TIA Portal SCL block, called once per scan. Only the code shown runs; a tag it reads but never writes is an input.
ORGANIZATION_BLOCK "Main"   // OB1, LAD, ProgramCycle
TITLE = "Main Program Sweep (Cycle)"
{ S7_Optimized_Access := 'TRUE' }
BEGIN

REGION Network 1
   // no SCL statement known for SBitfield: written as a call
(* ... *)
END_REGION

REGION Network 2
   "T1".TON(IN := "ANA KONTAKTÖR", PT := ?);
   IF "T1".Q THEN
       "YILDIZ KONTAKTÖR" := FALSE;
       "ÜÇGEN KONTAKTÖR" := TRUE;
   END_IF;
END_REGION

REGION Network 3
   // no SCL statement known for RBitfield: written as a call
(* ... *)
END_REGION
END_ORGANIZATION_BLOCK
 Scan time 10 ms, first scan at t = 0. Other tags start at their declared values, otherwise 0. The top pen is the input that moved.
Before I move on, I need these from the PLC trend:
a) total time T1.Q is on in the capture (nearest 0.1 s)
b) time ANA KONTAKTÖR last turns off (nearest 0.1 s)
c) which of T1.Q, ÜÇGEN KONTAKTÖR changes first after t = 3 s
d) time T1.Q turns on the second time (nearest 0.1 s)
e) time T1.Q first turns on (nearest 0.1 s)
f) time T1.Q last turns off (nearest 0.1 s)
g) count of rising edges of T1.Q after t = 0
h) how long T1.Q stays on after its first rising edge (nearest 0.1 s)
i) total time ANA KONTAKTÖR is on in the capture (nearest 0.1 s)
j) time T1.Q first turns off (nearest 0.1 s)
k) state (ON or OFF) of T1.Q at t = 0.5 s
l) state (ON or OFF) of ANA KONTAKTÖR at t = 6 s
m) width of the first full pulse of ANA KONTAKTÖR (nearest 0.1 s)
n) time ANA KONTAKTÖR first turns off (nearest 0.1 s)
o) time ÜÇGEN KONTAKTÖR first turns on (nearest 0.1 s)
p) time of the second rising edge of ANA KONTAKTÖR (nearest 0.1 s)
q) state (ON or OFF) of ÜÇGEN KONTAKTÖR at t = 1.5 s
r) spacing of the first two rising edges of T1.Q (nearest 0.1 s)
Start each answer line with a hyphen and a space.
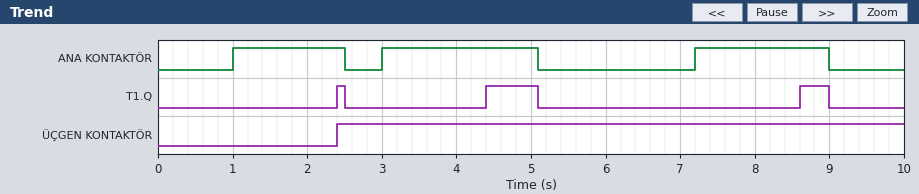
- 1.2 s
- 9.0 s
- T1.Q
- 4.4 s
- 2.4 s
- 9.0 s
- 3
- 0.1 s
- 5.4 s
- 2.5 s
- OFF
- OFF
- 1.5 s
- 2.5 s
- 2.4 s
- 3.0 s
- OFF
- 2.0 s
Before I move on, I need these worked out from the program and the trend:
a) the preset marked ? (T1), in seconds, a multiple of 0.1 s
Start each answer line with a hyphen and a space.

- 1.4 s
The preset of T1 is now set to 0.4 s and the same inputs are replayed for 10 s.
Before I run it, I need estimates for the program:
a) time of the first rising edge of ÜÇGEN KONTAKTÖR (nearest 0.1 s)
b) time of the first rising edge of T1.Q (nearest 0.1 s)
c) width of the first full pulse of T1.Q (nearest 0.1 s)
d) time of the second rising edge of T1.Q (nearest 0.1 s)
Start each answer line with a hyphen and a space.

- 1.4 s
- 1.4 s
- 1.1 s
- 3.4 s
